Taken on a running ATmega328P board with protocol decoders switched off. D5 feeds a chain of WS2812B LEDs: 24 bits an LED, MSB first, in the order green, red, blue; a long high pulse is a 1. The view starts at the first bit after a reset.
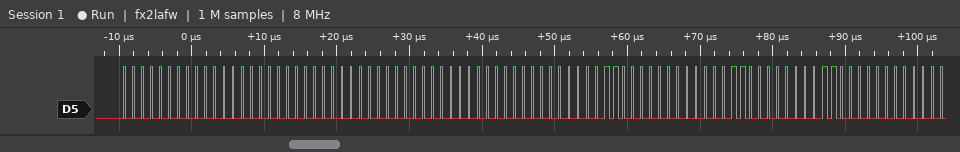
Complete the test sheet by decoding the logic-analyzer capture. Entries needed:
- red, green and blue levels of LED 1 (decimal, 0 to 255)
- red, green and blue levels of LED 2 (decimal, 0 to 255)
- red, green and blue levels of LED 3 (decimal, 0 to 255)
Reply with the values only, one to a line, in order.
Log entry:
0, 0, 0
0, 0, 0
0, 6, 24
